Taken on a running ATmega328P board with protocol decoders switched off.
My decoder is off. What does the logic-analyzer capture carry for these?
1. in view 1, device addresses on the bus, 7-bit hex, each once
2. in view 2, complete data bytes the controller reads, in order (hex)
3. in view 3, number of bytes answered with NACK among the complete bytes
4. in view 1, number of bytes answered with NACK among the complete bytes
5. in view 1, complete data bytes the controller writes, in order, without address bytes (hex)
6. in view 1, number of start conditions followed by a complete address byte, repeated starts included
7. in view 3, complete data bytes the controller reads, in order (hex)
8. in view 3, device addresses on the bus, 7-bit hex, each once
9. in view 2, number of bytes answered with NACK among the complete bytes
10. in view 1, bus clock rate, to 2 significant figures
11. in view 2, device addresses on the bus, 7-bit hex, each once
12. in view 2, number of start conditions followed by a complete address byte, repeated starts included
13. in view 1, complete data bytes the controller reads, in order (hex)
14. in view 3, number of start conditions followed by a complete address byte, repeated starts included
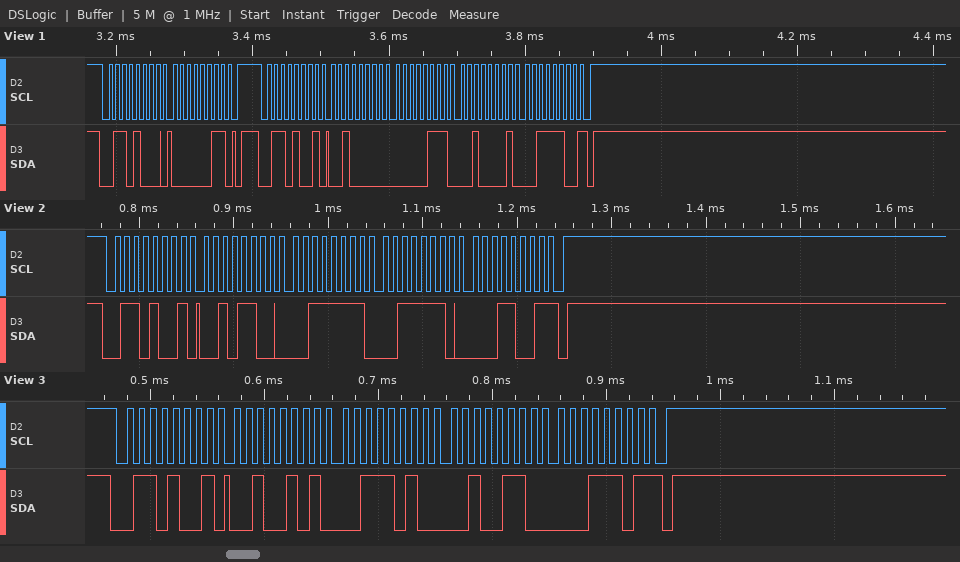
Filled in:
0x34
2C 3F 3E 19
1
1
03
2
25 3A 26 1D
0x34
1
100 kHz
0x34
1
20 07 21 3C
1
